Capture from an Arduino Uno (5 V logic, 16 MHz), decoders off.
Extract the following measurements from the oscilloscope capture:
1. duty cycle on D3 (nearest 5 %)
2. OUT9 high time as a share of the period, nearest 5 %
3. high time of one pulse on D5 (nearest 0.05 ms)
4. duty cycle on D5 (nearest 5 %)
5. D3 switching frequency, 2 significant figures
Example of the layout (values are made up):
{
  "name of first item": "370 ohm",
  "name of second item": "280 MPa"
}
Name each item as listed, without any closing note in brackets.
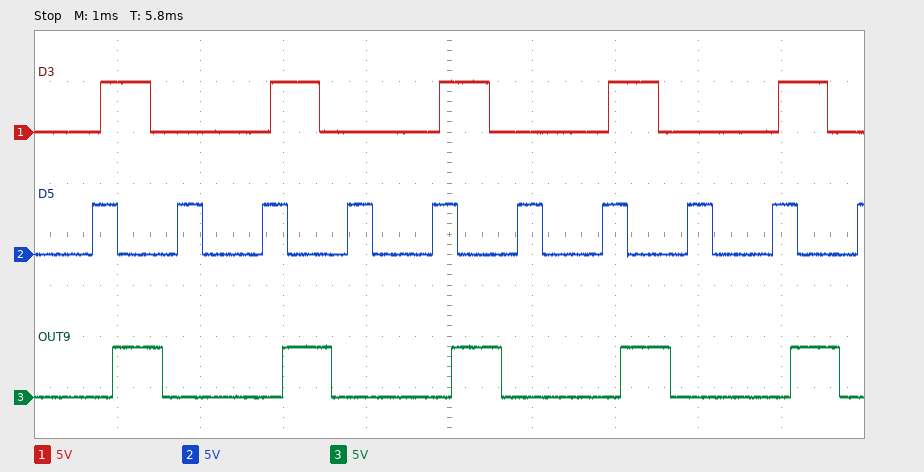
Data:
{
  "duty cycle on D3": "30 %",
  "OUT9 high time as a share of the period, nearest 5 %": "30 %",
  "high time of one pulse on D5": "0.30 ms",
  "duty cycle on D5": "30 %",
  "D3 switching frequency, 2 significant figures": "490 Hz"
}
